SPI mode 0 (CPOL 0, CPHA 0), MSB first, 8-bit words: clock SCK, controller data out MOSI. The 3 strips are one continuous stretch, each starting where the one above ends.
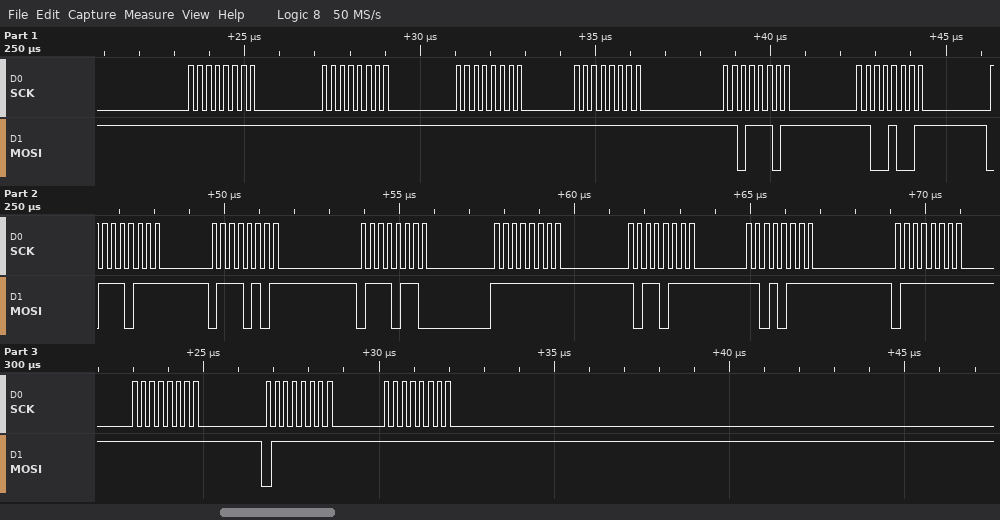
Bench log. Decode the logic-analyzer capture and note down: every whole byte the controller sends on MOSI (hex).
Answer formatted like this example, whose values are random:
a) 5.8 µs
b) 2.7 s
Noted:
a) FF FF FF FF DD C9 77 75 76 FF B7 D7 7F FF 7F FF
